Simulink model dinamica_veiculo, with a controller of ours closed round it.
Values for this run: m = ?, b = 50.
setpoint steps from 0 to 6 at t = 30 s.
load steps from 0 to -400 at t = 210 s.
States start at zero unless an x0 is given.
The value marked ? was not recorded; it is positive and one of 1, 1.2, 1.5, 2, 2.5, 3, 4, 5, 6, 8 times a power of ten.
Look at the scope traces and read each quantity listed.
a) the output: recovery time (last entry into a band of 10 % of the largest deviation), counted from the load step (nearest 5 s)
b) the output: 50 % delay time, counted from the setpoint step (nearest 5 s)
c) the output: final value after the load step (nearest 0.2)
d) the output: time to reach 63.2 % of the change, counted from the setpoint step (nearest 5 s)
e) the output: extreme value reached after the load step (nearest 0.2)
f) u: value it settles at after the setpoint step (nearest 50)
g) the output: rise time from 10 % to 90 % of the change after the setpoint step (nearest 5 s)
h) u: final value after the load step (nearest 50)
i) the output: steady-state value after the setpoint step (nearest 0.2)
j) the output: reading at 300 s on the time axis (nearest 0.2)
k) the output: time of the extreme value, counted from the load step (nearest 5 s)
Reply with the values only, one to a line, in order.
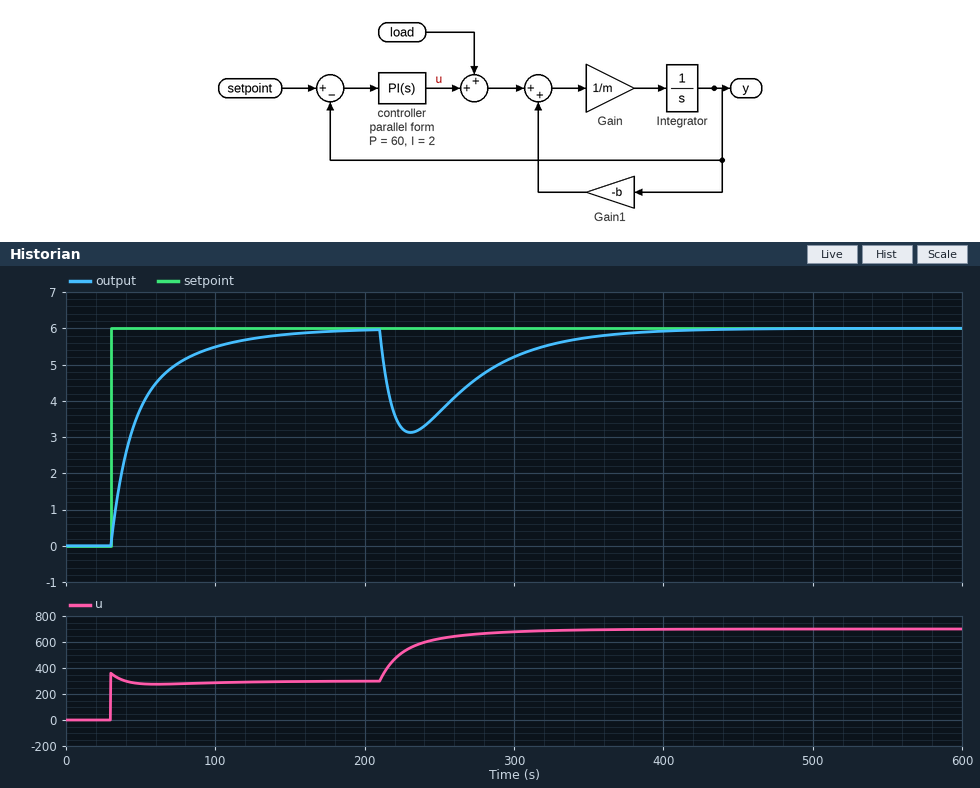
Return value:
135 s
15 s
6.0
20 s
3.2
300
60 s
700
6.0
5.2
20 s
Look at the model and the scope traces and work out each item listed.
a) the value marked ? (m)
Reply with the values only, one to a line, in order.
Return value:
1000
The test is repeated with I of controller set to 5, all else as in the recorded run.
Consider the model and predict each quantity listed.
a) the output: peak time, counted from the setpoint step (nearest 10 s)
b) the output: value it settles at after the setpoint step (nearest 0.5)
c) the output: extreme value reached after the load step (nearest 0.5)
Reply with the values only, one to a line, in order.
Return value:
50 s
6.0
3.5
